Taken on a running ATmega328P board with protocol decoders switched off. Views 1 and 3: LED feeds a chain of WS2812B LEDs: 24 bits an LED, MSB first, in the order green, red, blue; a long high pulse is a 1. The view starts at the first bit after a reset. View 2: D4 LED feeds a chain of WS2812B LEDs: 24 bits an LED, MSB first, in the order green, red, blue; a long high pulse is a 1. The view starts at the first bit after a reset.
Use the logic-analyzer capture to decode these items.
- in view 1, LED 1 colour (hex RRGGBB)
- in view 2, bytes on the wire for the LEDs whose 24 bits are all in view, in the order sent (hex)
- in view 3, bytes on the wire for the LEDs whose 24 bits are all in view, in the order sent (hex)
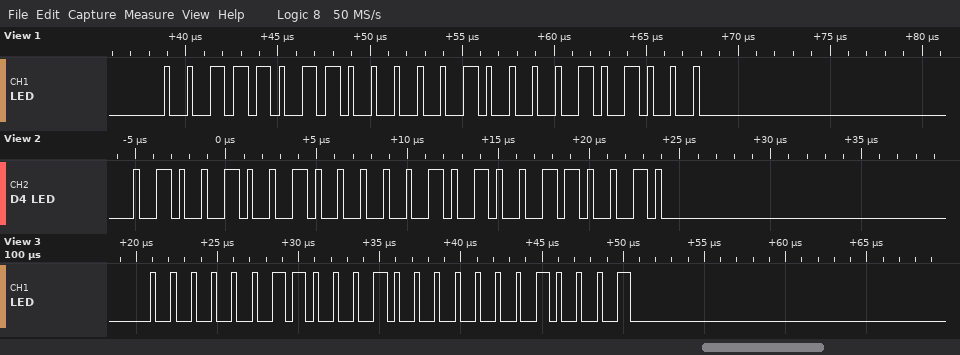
#043B28
49 05 32
03 10 11
